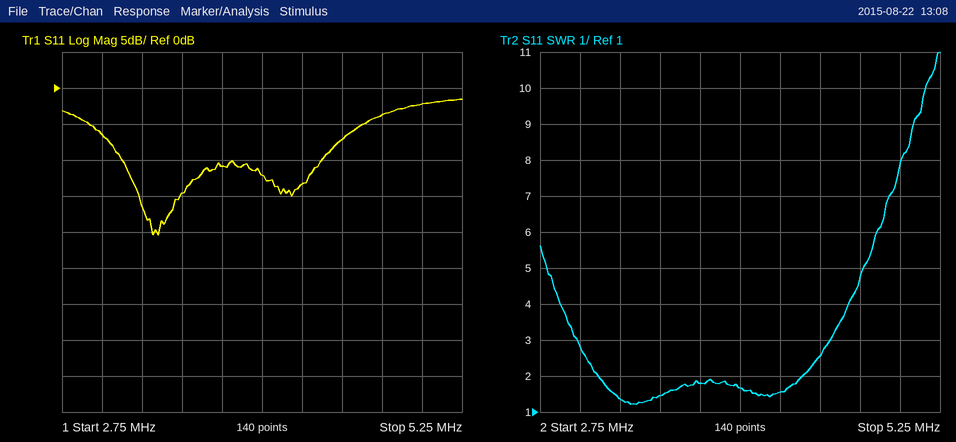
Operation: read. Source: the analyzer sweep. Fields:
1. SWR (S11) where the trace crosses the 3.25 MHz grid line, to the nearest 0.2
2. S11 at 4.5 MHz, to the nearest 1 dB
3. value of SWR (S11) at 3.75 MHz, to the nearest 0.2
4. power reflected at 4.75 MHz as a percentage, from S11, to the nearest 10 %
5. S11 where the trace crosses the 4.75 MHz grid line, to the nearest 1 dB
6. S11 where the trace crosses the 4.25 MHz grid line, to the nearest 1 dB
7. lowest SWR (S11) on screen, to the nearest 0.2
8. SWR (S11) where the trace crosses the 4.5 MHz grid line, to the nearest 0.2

1.4
-7 dB
1.8
40 %
-4 dB
-13 dB
1.2
2.6
